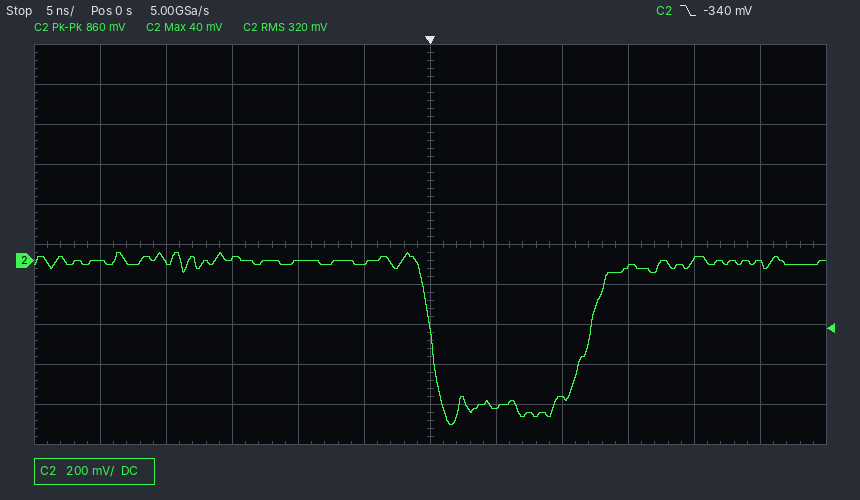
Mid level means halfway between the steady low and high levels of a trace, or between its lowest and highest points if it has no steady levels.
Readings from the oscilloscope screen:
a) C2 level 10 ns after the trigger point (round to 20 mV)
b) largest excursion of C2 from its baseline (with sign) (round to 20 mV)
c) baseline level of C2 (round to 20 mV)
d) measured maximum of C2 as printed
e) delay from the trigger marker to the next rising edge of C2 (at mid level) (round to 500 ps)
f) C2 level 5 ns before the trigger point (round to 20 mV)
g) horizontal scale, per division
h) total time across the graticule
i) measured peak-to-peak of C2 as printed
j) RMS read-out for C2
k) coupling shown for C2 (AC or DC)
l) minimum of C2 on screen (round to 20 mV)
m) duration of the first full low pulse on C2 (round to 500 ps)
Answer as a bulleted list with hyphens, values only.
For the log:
- -680 mV
- -800 mV
- -20 mV
- 40 mV
- 12.0 ns
- -20 mV
- 5 ns
- 60 ns
- 860 mV
- 320 mV
- DC
- -820 mV
- 12.0 ns
